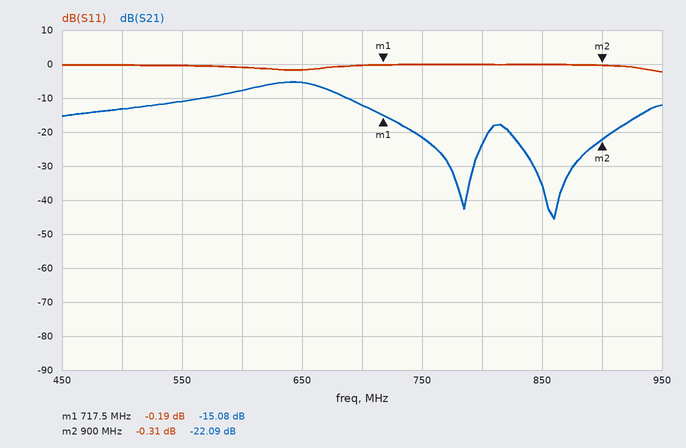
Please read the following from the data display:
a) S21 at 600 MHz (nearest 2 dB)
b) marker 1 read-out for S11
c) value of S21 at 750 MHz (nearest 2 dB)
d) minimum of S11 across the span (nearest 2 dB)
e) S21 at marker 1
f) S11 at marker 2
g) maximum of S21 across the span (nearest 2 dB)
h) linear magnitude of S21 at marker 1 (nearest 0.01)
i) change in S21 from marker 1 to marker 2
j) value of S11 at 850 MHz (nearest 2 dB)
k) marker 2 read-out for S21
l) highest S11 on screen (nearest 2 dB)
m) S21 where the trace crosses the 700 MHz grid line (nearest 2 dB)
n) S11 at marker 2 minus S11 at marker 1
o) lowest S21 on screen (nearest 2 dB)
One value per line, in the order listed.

-8 dB
-0.19 dB
-22 dB
-2 dB
-15.08 dB
-0.31 dB
-6 dB
0.18
-7.01 dB
0 dB
-22.09 dB
0 dB
-12 dB
-0.12 dB
-46 dB
